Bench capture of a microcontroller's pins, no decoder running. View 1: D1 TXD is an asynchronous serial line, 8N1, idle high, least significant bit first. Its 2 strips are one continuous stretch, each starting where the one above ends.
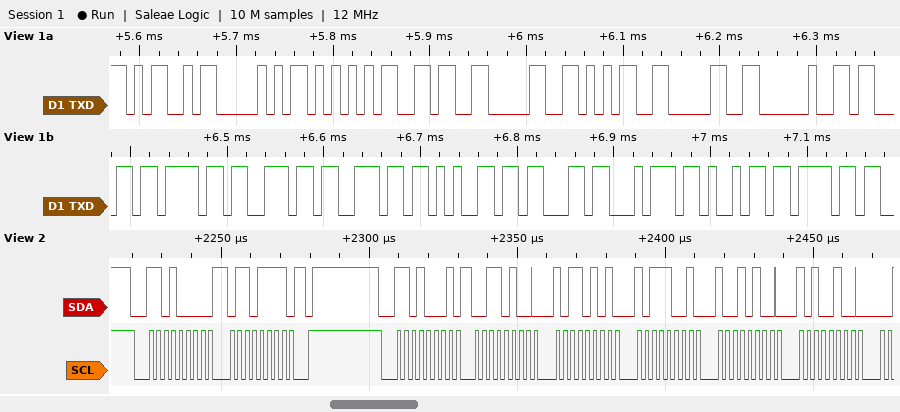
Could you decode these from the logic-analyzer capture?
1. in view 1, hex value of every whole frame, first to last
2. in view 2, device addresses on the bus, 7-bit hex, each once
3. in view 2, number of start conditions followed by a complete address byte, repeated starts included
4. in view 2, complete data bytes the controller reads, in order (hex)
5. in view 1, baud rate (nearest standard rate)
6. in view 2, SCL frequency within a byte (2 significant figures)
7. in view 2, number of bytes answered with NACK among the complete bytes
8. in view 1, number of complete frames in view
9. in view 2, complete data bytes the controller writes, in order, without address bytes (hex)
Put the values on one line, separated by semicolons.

4D 50 55 36 30 35 30 20 63 6F 6E 6E 65 63 74 69 6F; 0x68; 2; 34 B5 B9 94 A4; 115200 baud; 400 kHz; 0; 17; 6F
